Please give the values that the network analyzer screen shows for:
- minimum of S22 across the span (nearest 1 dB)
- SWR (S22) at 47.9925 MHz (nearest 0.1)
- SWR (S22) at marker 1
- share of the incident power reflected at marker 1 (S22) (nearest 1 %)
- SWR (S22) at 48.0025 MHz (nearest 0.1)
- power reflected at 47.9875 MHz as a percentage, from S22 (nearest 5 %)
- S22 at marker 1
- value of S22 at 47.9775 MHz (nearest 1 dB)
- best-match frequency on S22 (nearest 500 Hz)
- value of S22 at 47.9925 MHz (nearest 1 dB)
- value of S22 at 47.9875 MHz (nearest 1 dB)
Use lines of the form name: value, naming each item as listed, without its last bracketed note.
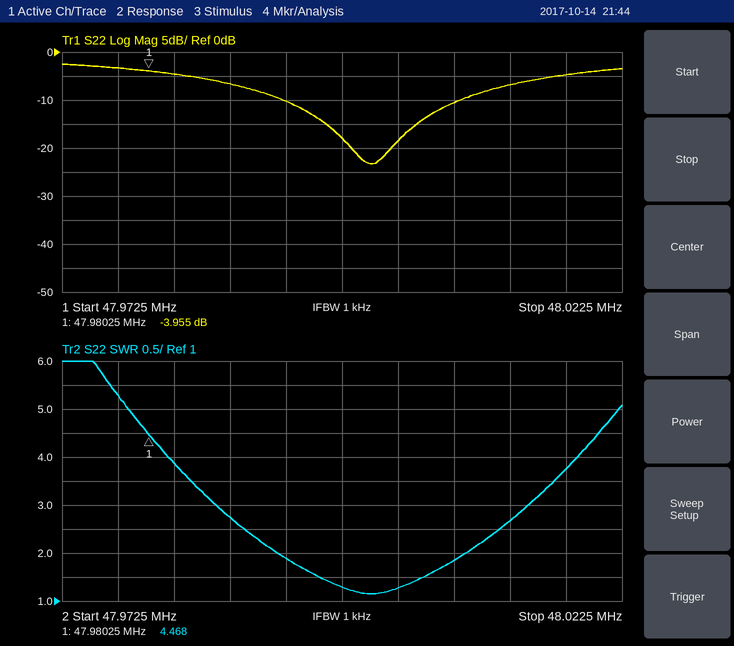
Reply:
minimum of S22 across the span: -23 dB
SWR (S22) at 47.9925 MHz: 1.9
SWR (S22) at marker 1: 4.468
share of the incident power reflected at marker 1 (S22): 40 %
SWR (S22) at 48.0025 MHz: 1.3
power reflected at 47.9875 MHz as a percentage, from S22: 20 %
S22 at marker 1: -3.955 dB
value of S22 at 47.9775 MHz: -3 dB
best-match frequency on S22: 48.0000 MHz
value of S22 at 47.9925 MHz: -10 dB
value of S22 at 47.9875 MHz: -7 dB
